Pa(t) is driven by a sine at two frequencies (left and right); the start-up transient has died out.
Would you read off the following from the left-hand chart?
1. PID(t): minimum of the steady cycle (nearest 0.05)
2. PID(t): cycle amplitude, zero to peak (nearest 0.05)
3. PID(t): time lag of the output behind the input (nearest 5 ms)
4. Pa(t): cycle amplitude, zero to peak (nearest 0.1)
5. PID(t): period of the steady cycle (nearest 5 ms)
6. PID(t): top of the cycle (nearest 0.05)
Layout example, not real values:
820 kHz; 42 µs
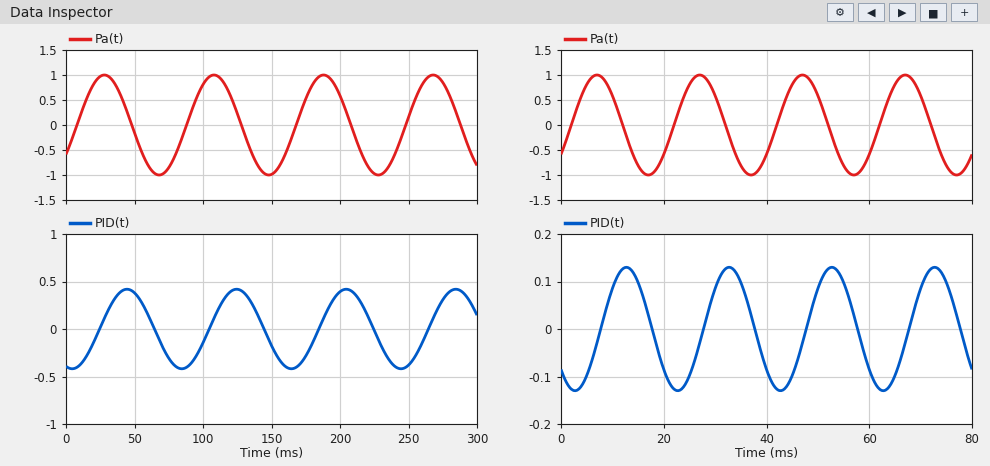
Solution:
-0.40; 0.40; 15 ms; 1.0; 80 ms; 0.40
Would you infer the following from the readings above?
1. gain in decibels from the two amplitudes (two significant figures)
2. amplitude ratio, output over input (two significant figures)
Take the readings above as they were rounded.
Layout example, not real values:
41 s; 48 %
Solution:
-8.0 dB; 0.40
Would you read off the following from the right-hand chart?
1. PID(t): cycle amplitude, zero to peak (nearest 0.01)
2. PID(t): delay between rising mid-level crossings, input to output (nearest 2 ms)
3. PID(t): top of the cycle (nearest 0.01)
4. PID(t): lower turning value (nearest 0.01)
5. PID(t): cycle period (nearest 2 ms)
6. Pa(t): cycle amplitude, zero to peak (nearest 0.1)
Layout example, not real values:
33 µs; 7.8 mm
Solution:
0.13; 6 ms; 0.13; -0.13; 20 ms; 1.0
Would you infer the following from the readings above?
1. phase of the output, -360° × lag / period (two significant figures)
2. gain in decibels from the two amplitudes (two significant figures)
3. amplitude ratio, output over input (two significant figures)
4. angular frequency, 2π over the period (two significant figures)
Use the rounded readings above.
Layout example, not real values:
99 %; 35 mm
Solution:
-110°; -18 dB; 0.13; 0.31 rad/ms
